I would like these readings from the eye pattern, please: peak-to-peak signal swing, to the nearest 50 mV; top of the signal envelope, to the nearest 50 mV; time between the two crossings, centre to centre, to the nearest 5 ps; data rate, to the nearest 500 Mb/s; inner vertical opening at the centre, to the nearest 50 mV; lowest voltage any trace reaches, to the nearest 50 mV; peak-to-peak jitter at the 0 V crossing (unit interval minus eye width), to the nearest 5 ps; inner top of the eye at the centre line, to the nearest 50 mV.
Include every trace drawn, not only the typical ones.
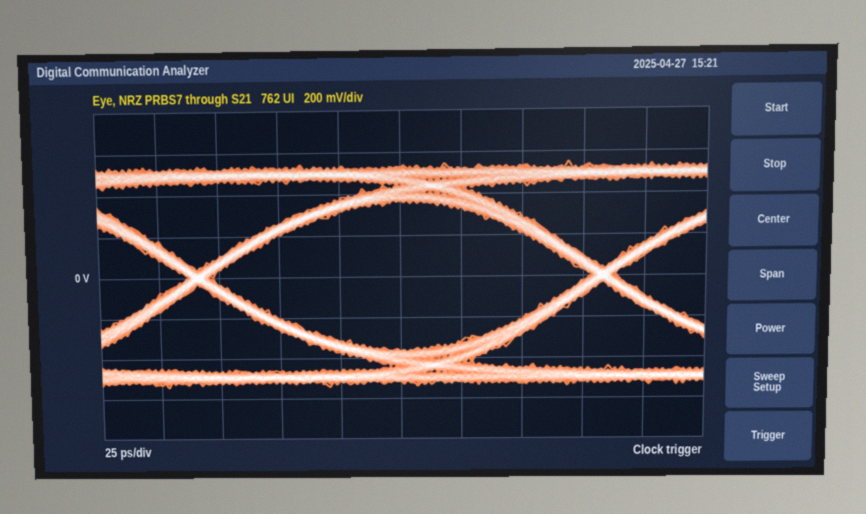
1.10 V
550 mV
165 ps
6.0 Gb/s
750 mV
-550 mV
10 ps
350 mV
